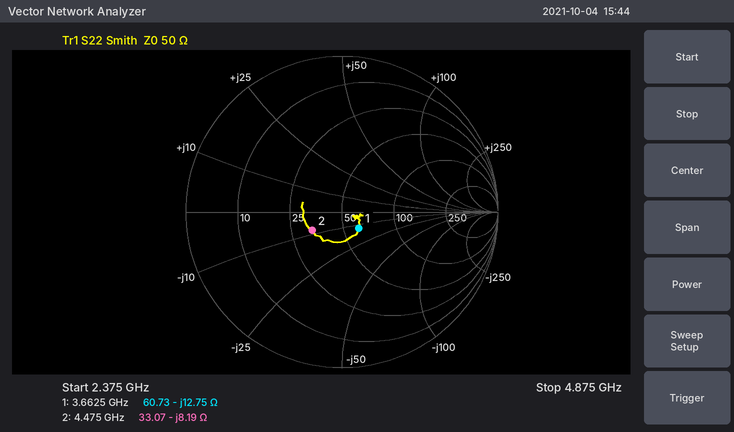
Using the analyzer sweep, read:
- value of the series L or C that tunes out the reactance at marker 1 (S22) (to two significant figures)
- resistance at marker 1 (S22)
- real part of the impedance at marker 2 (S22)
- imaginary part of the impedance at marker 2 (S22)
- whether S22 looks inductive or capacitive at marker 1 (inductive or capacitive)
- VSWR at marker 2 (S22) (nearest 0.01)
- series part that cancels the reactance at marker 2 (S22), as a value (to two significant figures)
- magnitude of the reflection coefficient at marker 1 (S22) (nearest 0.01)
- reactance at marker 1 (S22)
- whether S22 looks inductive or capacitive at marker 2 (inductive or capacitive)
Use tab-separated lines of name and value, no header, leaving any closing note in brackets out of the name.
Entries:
value of the series L or C that tunes out the reactance at marker 1 (S22)	550 pH
resistance at marker 1	60.73 Ω
real part of the impedance at marker 2	33.07 Ω
imaginary part of the impedance at marker 2	-8.19 Ω
whether S22 looks inductive or capacitive at marker 1	capacitive
VSWR at marker 2 (S22)	1.58
series part that cancels the reactance at marker 2 (S22), as a value	290 pH
magnitude of the reflection coefficient at marker 1 (S22)	0.15
reactance at marker 1	-12.75 Ω
whether S22 looks inductive or capacitive at marker 2	capacitive
